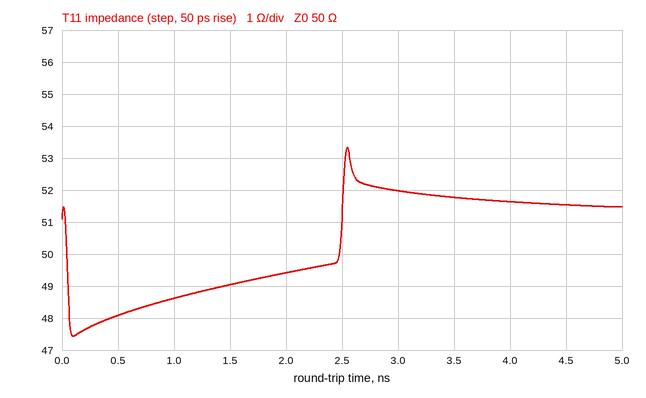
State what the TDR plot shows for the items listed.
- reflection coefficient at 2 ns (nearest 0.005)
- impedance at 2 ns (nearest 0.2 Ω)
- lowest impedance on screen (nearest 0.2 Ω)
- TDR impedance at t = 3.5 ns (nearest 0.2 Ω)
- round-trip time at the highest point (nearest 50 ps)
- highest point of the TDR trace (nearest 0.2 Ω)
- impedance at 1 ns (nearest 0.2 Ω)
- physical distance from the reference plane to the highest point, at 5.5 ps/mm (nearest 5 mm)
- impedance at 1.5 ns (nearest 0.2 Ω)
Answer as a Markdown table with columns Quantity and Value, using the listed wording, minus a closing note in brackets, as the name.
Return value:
| Quantity | Value |
|---|---|
| reflection coefficient at 2 ns | -0.005 |
| impedance at 2 ns | 49.4 Ω |
| lowest impedance on screen | 47.4 Ω |
| TDR impedance at t = 3.5 ns | 51.8 Ω |
| round-trip time at the highest point | 2.55 ns |
| highest point of the TDR trace | 53.4 Ω |
| impedance at 1 ns | 48.6 Ω |
| physical distance from the reference plane to the highest point, at 5.5 ps/mm | 230 mm |
| impedance at 1.5 ns | 49.0 Ω |
